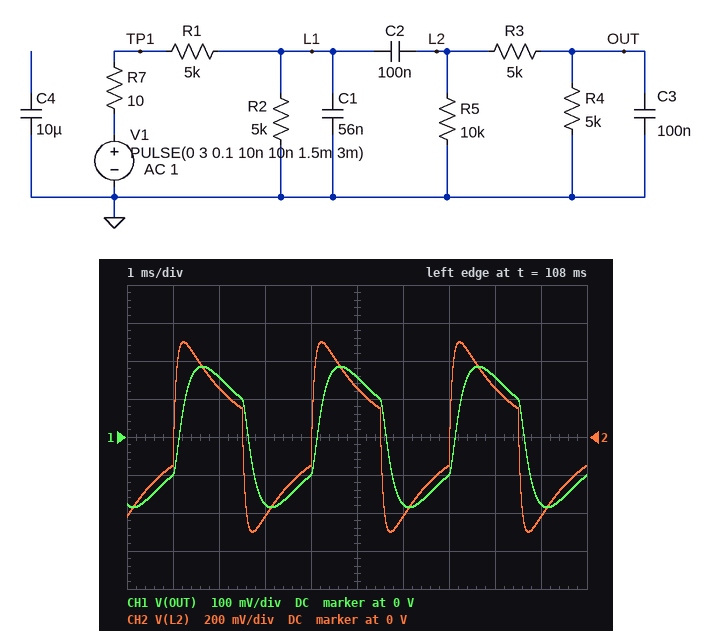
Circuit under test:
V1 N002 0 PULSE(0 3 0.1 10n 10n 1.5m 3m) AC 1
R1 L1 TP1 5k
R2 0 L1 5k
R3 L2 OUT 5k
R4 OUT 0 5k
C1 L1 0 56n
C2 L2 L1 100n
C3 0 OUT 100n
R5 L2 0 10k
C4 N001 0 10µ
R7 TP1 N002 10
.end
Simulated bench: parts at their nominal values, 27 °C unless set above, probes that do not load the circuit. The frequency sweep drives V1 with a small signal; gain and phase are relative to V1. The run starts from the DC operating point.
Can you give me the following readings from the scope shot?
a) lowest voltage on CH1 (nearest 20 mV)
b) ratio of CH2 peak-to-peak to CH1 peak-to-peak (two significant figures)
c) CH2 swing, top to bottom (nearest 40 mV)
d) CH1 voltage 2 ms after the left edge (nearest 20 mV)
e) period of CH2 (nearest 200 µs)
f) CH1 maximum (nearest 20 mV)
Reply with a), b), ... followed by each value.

a) -180 mV
b) 2.7
c) 1.00 V
d) 160 mV
e) 3.0 ms
f) 180 mV
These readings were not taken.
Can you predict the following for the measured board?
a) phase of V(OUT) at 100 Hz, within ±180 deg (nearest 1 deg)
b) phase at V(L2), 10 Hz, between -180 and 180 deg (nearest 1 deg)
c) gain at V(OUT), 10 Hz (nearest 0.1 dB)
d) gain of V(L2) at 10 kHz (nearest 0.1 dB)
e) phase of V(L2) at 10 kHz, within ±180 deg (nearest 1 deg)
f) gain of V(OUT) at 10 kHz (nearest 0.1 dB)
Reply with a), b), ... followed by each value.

a) 48 deg
b) 86 deg
c) -42.1 dB
d) -25.2 dB
e) -76 deg
f) -55.1 dB
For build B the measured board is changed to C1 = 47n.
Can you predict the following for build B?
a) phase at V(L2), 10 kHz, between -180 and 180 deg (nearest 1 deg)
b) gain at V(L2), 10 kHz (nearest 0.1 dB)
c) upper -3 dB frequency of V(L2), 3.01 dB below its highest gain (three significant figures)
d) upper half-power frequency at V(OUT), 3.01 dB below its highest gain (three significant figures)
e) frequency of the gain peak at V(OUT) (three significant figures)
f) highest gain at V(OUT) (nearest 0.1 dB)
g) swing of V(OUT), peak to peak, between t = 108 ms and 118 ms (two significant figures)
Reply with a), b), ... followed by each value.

a) -74 deg
b) -23.7 dB
c) 2.80 kHz
d) 815 Hz
e) 311 Hz
f) -19.6 dB
g) 380 mV
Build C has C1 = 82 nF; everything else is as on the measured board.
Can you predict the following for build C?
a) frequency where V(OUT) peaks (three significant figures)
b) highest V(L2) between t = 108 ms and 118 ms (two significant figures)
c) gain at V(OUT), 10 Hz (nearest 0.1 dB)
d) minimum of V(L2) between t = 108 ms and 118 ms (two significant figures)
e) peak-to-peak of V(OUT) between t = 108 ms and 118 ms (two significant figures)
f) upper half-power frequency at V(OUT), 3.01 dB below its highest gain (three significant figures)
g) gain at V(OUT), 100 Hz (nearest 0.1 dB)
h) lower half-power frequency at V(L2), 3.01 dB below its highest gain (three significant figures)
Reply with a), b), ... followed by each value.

a) 287 Hz
b) 440 mV
c) -42.1 dB
d) -440 mV
e) 350 mV
f) 722 Hz
g) -23.6 dB
h) 128 Hz
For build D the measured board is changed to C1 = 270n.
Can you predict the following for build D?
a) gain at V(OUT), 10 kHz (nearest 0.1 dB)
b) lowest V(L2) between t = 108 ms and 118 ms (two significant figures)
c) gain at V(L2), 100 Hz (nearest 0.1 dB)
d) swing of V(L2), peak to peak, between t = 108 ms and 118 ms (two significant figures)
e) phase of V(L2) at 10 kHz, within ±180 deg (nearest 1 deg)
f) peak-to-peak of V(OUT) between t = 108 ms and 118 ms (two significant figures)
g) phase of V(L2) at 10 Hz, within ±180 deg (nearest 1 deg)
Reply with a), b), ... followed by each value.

a) -68.6 dB
b) -250 mV
c) -18.3 dB
d) 500 mV
e) -85 deg
f) 230 mV
g) 84 deg
